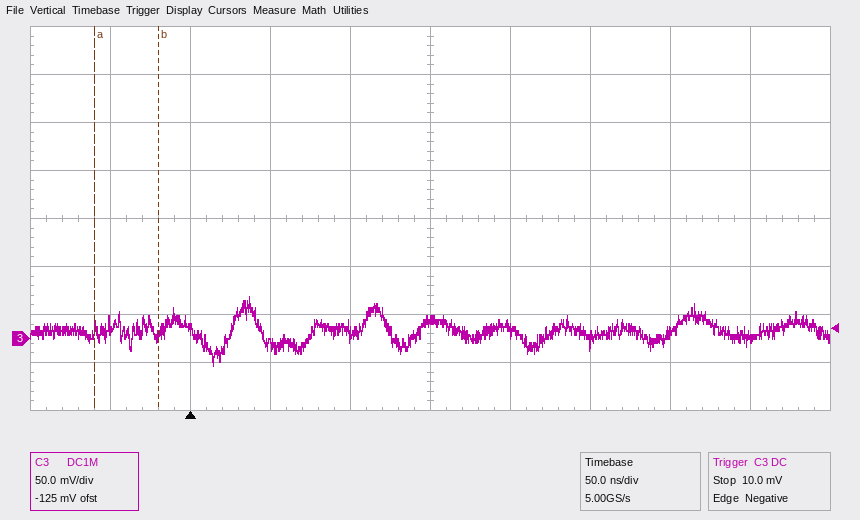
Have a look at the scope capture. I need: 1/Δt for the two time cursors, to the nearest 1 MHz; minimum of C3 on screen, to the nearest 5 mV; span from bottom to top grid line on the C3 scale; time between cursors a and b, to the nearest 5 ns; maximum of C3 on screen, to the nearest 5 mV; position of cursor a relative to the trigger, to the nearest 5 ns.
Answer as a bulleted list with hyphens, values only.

- 25 MHz
- -30 mV
- 400 mV
- 40 ns
- 45 mV
- -60 ns
